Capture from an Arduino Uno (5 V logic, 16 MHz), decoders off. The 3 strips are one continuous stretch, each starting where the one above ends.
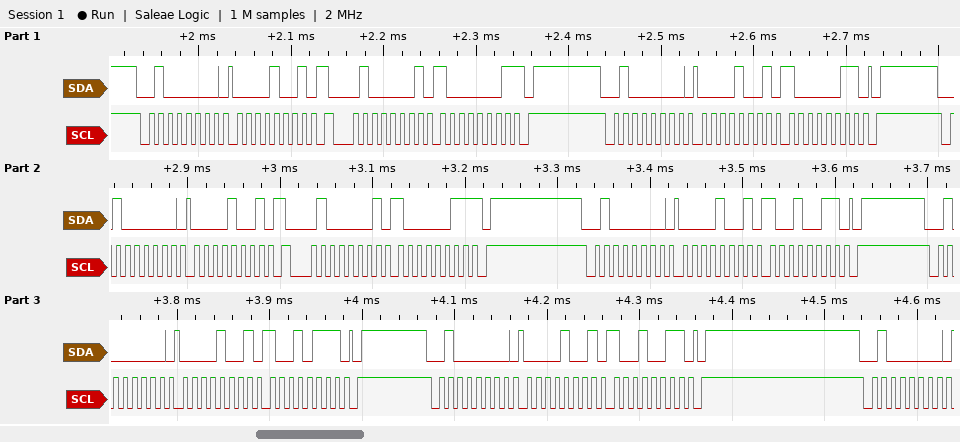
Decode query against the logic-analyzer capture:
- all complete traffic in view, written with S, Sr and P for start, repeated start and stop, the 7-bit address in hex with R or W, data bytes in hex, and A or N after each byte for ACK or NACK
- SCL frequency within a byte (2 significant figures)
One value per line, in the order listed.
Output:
S 20W A 09 A Sr 20R A 81 N P S 20W A 09 A 83 A P S 20W A 09 A Sr 20R A 83 N P S 20W A 09 A 93 A P S 20W A 09 A 97 A P S 20W A 09 A 93 A P S 20W A
100 kHz
